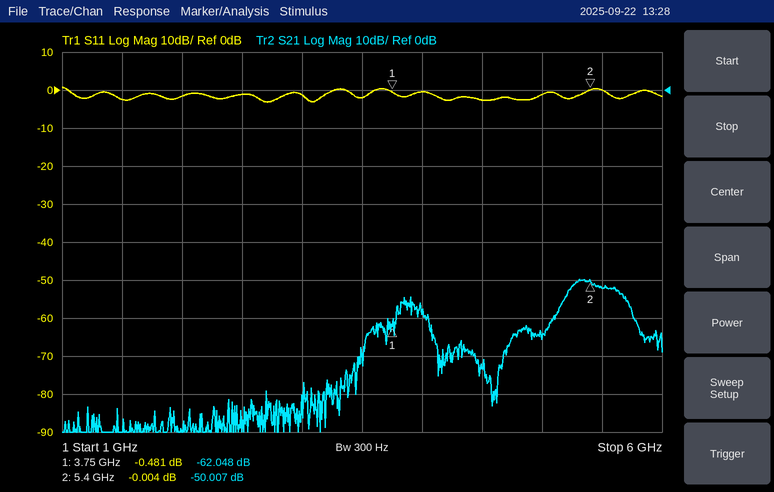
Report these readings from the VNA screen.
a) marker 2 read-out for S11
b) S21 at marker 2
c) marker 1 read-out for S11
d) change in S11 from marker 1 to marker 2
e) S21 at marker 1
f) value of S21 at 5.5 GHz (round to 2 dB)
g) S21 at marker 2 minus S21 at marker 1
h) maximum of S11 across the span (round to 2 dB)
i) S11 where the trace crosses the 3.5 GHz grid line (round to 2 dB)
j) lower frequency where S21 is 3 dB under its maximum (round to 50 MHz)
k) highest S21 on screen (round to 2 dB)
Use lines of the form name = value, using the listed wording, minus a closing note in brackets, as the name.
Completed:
marker 2 read-out for S11 = -0.004 dB
S21 at marker 2 = -50.007 dB
marker 1 read-out for S11 = -0.481 dB
change in S11 from marker 1 to marker 2 = 0.477 dB
S21 at marker 1 = -62.048 dB
value of S21 at 5.5 GHz = -52 dB
S21 at marker 2 minus S21 at marker 1 = 12.041 dB
maximum of S11 across the span = 0 dB
S11 where the trace crosses the 3.5 GHz grid line = -2 dB
lower frequency where S21 is 3 dB under its maximum = 5.20 GHz
highest S21 on screen = -50 dB
